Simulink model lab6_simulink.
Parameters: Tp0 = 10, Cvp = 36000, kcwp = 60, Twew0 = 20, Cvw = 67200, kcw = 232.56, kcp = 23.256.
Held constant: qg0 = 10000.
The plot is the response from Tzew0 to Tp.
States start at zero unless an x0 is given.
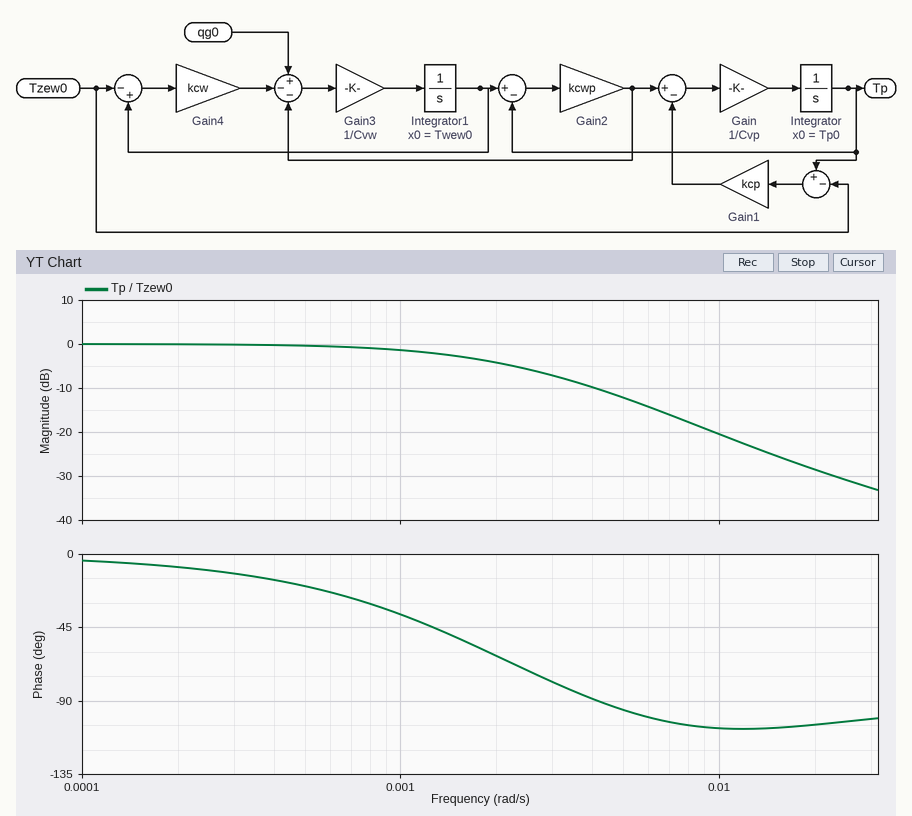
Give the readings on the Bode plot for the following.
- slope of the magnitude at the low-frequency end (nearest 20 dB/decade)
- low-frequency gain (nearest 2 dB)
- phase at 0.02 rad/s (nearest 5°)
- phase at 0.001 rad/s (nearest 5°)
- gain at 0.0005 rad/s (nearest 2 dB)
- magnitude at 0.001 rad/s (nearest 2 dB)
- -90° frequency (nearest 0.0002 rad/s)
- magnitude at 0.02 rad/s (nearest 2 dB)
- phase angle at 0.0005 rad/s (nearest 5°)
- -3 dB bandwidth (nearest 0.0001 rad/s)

0 dB/decade
0 dB
-105°
-35°
0 dB
-2 dB
0.0042 rad/s
-28 dB
-20°
0.0016 rad/s
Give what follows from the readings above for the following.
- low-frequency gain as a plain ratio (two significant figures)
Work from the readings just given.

1.0
